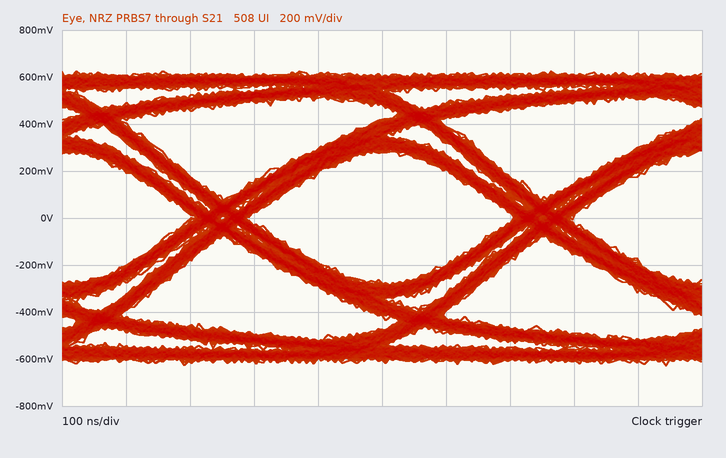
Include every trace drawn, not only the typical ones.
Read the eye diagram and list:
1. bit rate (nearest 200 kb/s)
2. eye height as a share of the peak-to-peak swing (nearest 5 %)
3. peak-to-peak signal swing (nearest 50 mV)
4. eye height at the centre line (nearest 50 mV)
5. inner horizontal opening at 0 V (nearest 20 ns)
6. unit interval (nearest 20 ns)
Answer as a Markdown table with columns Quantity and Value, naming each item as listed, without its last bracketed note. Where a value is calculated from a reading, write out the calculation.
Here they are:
| Quantity | Value |
|---|---|
| bit rate | 2.0 Mb/s |
| eye height as a share of the peak-to-peak swing | 550 mV / 1.25 V ≈ 44.0 %, so 45 % to the nearest 5 % |
| peak-to-peak signal swing | 1.25 V |
| eye height at the centre line | 550 mV |
| inner horizontal opening at 0 V | 420 ns |
| unit interval | 500 ns |
